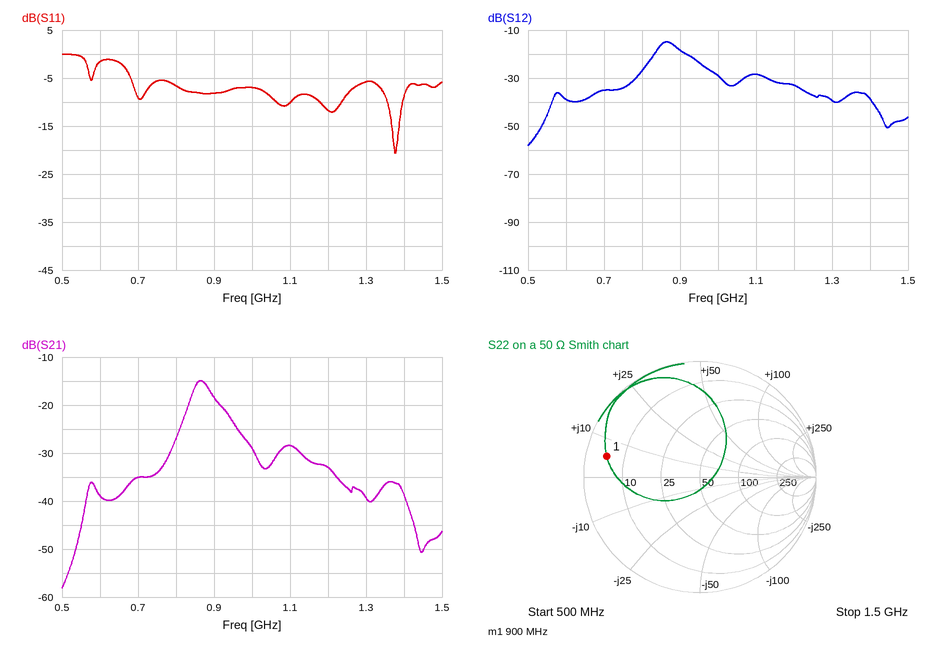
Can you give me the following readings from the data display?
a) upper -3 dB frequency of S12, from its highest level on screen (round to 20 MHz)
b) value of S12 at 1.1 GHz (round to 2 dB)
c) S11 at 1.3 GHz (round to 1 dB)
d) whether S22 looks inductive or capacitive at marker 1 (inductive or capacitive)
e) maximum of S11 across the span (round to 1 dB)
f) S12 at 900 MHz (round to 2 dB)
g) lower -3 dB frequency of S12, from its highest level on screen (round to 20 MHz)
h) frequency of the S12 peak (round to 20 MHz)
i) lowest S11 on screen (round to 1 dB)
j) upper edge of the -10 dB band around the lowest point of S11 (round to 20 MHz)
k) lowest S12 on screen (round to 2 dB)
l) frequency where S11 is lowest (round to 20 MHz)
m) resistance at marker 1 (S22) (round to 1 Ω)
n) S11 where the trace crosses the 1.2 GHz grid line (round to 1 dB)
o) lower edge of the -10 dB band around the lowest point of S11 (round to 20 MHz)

900 MHz
-28 dB
-6 dB
inductive
0 dB
-18 dB
840 MHz
860 MHz
-21 dB
1.40 GHz
-58 dB
1.38 GHz
5 Ω
-12 dB
1.36 GHz
